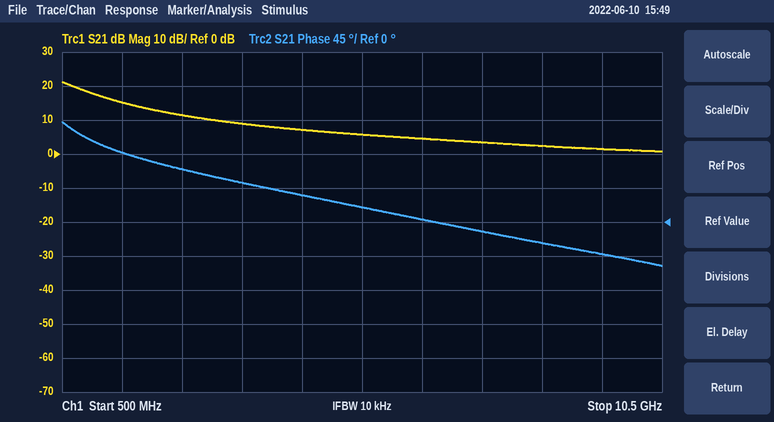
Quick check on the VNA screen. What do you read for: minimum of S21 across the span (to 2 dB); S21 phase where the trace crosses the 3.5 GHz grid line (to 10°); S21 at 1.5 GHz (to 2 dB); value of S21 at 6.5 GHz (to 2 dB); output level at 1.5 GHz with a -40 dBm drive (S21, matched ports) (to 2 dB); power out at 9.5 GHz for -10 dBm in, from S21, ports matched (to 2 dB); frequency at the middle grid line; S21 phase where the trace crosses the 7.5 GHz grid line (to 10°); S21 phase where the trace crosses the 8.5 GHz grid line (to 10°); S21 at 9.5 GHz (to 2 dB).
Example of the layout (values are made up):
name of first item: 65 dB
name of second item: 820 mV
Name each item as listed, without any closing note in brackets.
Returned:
minimum of S21 across the span: 0 dB
S21 phase where the trace crosses the 3.5 GHz grid line: 50°
S21 at 1.5 GHz: 16 dB
value of S21 at 6.5 GHz: 4 dB
output level at 1.5 GHz with a -40 dBm drive (S21, matched ports): -24 dBm
power out at 9.5 GHz for -10 dBm in, from S21, ports matched: -8 dBm
frequency at the middle grid line: 5.5 GHz
S21 phase where the trace crosses the 7.5 GHz grid line: -10°
S21 phase where the trace crosses the 8.5 GHz grid line: -30°
S21 at 9.5 GHz: 2 dB
